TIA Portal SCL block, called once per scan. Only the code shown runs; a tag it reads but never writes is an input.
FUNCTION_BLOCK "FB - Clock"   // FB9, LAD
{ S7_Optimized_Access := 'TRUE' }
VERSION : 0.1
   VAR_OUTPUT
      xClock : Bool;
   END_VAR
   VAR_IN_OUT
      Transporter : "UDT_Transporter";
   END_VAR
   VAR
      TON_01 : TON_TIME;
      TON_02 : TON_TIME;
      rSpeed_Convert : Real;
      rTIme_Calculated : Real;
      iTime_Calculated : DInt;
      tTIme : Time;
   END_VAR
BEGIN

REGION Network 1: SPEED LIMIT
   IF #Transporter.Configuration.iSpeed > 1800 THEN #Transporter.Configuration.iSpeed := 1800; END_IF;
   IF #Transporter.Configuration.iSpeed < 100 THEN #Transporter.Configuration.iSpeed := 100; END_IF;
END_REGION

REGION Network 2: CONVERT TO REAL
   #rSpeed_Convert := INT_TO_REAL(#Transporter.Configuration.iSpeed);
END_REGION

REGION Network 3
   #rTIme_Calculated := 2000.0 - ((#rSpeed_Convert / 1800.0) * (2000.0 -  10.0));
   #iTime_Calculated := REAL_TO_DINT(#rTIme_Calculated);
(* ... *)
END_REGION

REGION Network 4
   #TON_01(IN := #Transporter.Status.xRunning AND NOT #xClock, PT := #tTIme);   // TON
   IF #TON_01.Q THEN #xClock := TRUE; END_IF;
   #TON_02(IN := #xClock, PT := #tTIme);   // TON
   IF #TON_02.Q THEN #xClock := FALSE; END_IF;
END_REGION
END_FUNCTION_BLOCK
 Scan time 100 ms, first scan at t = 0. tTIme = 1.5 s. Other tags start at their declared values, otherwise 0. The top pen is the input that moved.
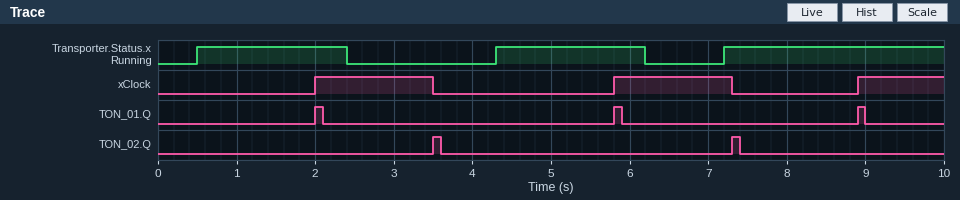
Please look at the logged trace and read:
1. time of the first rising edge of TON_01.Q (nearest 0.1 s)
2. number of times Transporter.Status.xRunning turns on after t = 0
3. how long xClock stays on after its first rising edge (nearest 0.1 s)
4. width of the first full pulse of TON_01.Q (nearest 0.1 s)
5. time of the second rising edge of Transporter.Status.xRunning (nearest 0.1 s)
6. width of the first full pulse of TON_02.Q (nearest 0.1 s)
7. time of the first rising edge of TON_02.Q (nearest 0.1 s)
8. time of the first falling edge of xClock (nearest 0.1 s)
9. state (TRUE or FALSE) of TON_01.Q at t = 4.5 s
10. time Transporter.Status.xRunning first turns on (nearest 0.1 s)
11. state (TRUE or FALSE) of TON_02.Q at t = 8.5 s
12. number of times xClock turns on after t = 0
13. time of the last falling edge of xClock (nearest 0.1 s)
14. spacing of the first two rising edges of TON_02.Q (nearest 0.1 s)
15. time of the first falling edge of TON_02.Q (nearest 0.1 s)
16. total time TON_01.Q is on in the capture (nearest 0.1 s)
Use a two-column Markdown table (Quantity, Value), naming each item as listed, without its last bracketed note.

| Quantity | Value |
|---|---|
| time of the first rising edge of TON_01.Q | 2.0 s |
| number of times Transporter.Status.xRunning turns on after t = 0 | 3 |
| how long xClock stays on after its first rising edge | 1.5 s |
| width of the first full pulse of TON_01.Q | 0.1 s |
| time of the second rising edge of Transporter.Status.xRunning | 4.3 s |
| width of the first full pulse of TON_02.Q | 0.1 s |
| time of the first rising edge of TON_02.Q | 3.5 s |
| time of the first falling edge of xClock | 3.5 s |
| state (TRUE or FALSE) of TON_01.Q at t = 4.5 s | FALSE |
| time Transporter.Status.xRunning first turns on | 0.5 s |
| state (TRUE or FALSE) of TON_02.Q at t = 8.5 s | FALSE |
| number of times xClock turns on after t = 0 | 3 |
| time of the last falling edge of xClock | 7.3 s |
| spacing of the first two rising edges of TON_02.Q | 3.8 s |
| time of the first falling edge of TON_02.Q | 3.6 s |
| total time TON_01.Q is on in the capture | 0.3 s |
